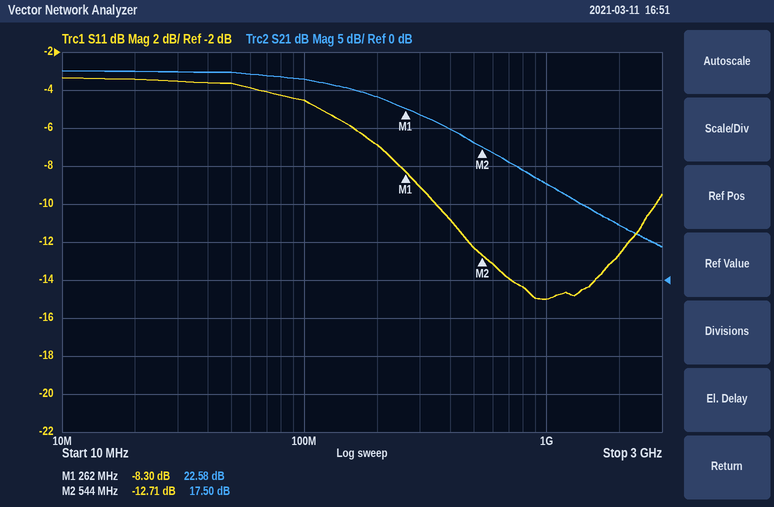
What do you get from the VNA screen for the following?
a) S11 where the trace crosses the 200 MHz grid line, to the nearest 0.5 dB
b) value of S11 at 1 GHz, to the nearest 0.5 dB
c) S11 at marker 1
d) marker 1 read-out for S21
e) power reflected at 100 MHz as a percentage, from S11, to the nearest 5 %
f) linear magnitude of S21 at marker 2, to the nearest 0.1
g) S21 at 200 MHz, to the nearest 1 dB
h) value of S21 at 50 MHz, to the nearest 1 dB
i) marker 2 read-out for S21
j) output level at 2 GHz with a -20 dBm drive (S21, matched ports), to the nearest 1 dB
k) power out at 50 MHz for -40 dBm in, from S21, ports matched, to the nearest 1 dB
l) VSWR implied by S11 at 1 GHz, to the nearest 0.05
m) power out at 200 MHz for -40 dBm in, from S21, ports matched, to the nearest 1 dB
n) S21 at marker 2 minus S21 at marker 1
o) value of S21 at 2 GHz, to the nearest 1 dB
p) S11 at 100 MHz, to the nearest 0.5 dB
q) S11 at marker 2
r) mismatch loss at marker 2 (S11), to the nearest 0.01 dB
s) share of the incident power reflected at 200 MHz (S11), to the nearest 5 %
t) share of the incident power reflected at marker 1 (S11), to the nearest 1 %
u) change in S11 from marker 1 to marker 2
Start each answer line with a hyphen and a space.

- -7.0 dB
- -15.0 dB
- -8.30 dB
- 22.58 dB
- 35 %
- 7.5
- 24 dB
- 27 dB
- 17.50 dB
- -13 dBm
- -13 dBm
- 1.45
- -16 dBm
- -5.08 dB
- 7 dB
- -4.5 dB
- -12.71 dB
- 0.24 dB
- 20 %
- 15 %
- -4.41 dB
